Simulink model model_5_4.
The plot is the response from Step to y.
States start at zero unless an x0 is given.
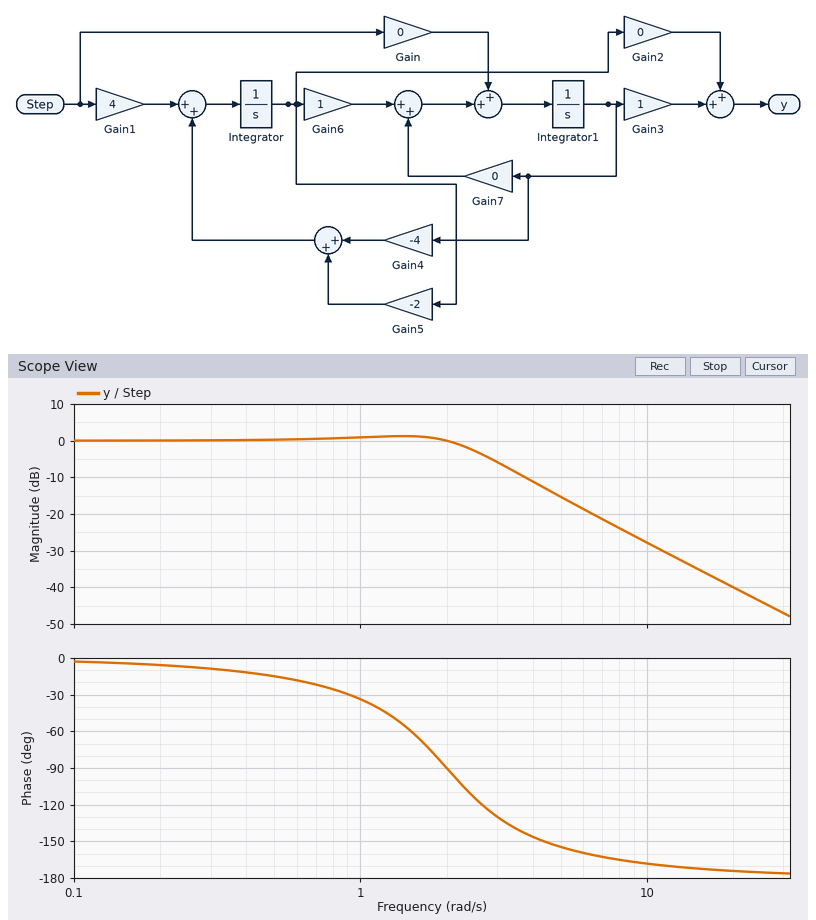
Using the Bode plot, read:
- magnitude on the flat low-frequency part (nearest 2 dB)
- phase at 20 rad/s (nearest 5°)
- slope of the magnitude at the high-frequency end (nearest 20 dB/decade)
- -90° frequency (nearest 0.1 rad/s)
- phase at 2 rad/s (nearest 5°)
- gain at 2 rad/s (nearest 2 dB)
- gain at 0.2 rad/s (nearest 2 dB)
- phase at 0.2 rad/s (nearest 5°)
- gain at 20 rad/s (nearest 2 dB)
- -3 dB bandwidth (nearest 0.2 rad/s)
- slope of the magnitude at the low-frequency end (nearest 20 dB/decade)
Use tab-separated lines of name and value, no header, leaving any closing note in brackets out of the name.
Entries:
magnitude on the flat low-frequency part	0 dB
phase at 20 rad/s	-175°
slope of the magnitude at the high-frequency end	-40 dB/decade
-90° frequency	2.0 rad/s
phase at 2 rad/s	-90°
gain at 2 rad/s	0 dB
gain at 0.2 rad/s	0 dB
phase at 0.2 rad/s	-5°
gain at 20 rad/s	-40 dB
-3 dB bandwidth	2.6 rad/s
slope of the magnitude at the low-frequency end	0 dB/decade
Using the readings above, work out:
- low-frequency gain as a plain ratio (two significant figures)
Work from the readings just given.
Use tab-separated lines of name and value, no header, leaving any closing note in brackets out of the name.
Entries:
low-frequency gain as a plain ratio	1.0
